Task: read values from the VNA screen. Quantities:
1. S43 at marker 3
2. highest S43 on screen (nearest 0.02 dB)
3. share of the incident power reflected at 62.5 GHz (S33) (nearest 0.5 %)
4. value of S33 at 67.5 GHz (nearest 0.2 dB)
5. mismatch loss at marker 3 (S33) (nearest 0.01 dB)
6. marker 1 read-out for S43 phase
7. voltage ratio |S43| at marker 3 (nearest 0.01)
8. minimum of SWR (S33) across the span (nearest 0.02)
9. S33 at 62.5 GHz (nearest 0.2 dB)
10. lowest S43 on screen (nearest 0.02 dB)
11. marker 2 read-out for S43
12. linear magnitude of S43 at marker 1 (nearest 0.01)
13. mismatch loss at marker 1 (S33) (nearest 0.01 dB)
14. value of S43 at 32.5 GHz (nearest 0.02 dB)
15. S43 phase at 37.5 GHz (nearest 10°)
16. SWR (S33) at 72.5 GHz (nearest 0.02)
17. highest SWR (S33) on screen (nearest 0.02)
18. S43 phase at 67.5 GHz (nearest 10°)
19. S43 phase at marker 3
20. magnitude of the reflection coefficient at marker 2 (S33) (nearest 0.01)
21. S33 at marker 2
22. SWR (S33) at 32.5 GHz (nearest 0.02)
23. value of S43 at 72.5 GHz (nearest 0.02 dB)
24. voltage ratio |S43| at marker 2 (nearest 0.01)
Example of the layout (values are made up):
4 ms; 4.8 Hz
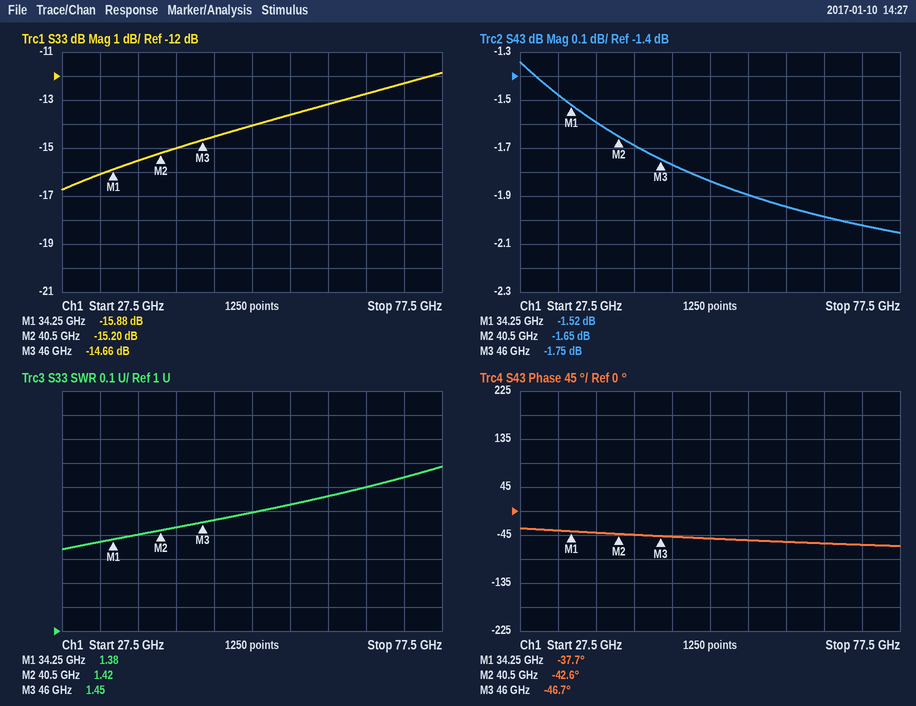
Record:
-1.75 dB; -1.34 dB; 5.0 %; -12.8 dB; 0.15 dB; -37.7°; 0.82; 1.34; -13.2 dB; -2.06 dB; -1.65 dB; 0.84; 0.11 dB; -1.48 dB; -40°; 1.64; 1.68; -60°; -46.7°; 0.17; -15.20 dB; 1.38; -2.02 dB; 0.83
